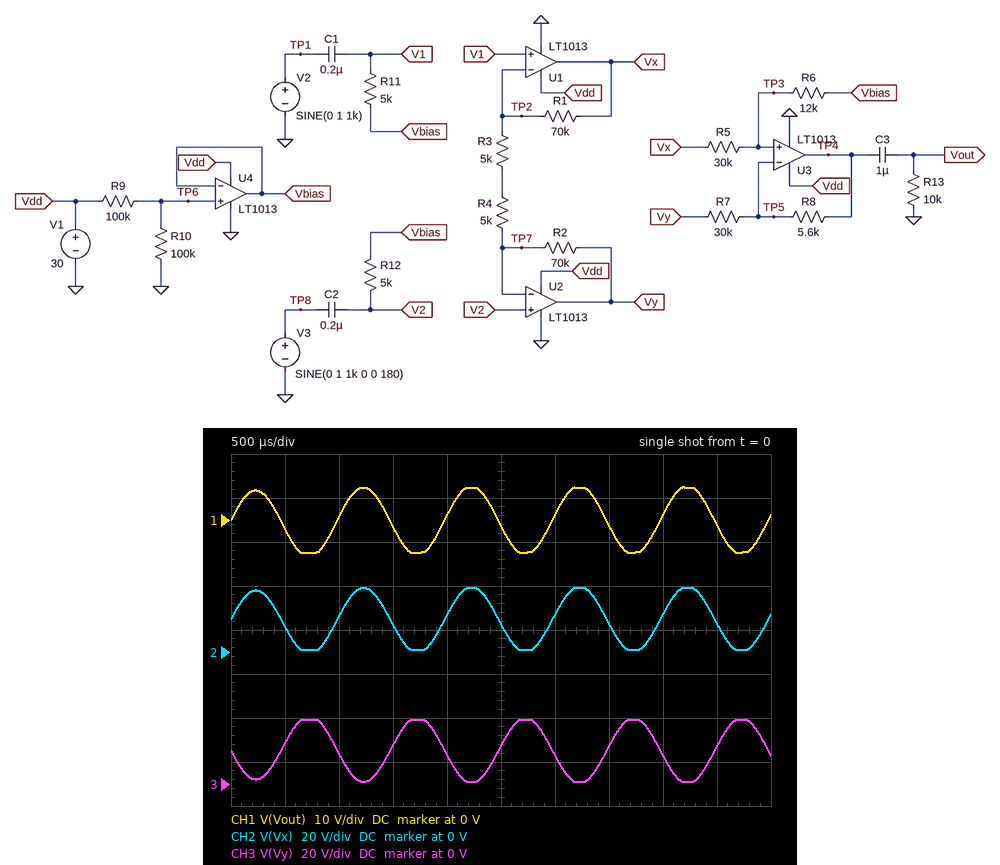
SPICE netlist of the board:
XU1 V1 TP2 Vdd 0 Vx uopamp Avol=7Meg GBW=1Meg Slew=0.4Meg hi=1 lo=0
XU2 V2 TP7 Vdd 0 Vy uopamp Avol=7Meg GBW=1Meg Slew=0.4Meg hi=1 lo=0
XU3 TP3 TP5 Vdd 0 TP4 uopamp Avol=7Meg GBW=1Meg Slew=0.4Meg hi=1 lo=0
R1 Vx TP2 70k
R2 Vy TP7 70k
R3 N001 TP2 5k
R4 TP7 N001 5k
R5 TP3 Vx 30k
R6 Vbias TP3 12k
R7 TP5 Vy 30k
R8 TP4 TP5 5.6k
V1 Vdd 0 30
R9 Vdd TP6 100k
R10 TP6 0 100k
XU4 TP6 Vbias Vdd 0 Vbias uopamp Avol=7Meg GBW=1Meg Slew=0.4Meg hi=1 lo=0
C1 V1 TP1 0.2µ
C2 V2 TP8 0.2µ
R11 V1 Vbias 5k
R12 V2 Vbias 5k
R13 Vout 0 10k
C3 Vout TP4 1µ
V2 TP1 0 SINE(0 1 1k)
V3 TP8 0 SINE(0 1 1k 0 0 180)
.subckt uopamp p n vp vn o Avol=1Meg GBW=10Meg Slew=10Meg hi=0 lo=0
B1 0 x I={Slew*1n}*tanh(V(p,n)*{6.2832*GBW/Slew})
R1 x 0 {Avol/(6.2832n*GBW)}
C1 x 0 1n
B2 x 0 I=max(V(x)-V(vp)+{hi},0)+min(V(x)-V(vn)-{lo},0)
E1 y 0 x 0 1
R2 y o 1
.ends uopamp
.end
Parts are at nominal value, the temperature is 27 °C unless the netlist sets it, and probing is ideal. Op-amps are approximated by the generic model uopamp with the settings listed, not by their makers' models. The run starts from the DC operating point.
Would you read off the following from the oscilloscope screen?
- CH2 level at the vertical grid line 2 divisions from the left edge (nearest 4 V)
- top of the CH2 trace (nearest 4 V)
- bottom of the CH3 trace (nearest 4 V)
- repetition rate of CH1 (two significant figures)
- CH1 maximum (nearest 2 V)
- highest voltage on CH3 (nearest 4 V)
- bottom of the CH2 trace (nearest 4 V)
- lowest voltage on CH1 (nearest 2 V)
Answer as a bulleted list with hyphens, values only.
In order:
- 16 V
- 28 V
- 0 V
- 1.0 kHz
- 8 V
- 28 V
- 0 V
- -8 V
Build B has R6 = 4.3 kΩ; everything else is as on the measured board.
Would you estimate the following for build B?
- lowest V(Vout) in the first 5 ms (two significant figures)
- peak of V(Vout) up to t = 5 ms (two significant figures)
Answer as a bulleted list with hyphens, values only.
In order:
- -4.8 V
- 4.7 V
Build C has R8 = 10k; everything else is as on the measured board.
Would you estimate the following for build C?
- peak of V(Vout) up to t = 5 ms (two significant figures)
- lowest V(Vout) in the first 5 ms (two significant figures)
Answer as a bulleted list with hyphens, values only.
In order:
- 10 V
- -10 V
